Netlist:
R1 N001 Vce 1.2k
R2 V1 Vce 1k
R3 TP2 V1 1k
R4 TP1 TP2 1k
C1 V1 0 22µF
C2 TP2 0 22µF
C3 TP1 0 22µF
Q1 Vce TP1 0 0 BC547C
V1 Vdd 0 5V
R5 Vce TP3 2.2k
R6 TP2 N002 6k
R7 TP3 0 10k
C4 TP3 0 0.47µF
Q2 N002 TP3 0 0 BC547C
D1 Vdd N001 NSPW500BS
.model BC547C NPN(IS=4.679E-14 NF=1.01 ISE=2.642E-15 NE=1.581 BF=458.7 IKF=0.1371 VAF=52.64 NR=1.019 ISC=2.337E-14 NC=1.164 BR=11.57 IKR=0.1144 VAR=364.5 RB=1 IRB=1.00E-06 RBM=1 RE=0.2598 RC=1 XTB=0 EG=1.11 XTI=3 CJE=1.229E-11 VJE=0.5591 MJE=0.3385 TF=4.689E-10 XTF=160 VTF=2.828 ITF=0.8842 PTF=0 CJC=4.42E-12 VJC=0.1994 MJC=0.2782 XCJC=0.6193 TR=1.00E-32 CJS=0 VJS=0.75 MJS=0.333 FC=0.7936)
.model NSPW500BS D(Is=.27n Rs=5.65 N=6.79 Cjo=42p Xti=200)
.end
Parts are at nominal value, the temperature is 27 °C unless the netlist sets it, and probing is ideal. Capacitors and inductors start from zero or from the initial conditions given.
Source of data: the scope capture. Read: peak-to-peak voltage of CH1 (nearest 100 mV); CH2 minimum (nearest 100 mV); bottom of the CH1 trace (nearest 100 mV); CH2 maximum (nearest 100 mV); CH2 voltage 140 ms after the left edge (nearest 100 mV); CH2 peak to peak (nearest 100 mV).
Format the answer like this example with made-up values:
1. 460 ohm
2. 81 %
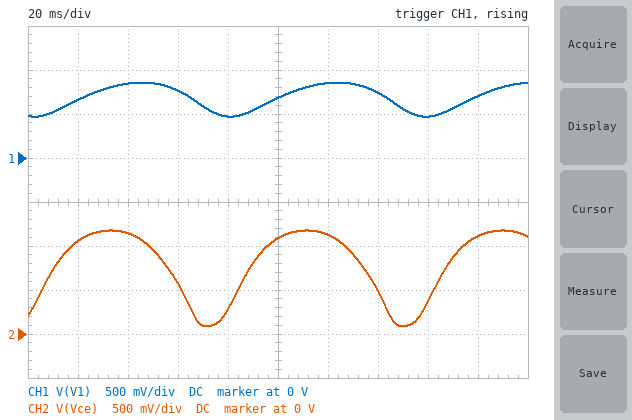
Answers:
1. 400 mV
2. 100 mV
3. 500 mV
4. 1.2 V
5. 500 mV
6. 1.1 V
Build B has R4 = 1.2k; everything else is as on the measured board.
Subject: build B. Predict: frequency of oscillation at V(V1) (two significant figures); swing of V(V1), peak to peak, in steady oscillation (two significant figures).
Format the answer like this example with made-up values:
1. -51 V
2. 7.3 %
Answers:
1. 12 Hz
2. 400 mV
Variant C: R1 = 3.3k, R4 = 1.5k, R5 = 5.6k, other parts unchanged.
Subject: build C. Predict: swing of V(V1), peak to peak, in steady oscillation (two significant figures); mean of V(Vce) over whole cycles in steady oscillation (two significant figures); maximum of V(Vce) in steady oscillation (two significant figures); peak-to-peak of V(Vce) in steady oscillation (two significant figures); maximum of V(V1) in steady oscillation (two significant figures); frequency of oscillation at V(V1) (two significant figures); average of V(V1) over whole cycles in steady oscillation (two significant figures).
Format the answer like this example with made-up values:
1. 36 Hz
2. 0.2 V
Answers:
1. 270 mV
2. 670 mV
3. 910 mV
4. 690 mV
5. 740 mV
6. 9.1 Hz
7. 630 mV
